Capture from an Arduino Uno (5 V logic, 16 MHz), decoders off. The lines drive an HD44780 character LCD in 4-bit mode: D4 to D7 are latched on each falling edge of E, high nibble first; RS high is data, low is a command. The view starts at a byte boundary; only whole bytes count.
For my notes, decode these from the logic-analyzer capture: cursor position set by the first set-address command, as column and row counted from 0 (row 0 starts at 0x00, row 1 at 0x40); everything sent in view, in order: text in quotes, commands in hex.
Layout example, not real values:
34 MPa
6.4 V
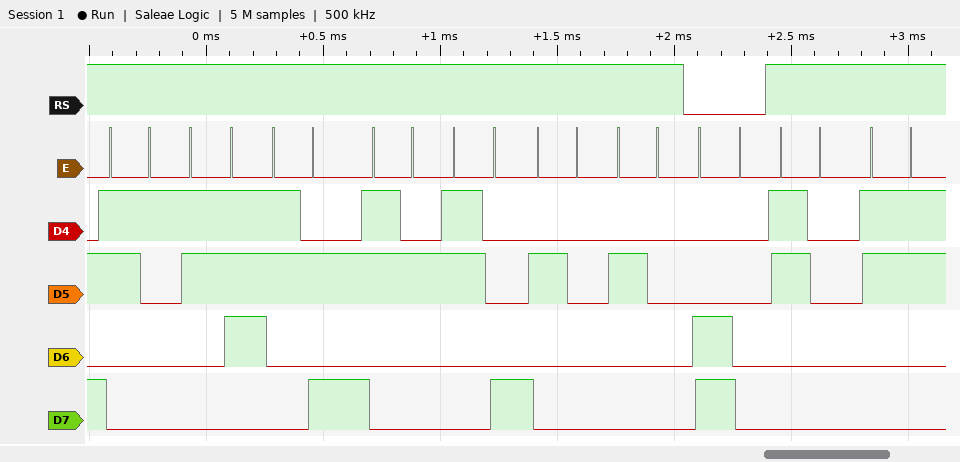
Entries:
column 0, row 1
"17:28  " 0xC0 "03"
